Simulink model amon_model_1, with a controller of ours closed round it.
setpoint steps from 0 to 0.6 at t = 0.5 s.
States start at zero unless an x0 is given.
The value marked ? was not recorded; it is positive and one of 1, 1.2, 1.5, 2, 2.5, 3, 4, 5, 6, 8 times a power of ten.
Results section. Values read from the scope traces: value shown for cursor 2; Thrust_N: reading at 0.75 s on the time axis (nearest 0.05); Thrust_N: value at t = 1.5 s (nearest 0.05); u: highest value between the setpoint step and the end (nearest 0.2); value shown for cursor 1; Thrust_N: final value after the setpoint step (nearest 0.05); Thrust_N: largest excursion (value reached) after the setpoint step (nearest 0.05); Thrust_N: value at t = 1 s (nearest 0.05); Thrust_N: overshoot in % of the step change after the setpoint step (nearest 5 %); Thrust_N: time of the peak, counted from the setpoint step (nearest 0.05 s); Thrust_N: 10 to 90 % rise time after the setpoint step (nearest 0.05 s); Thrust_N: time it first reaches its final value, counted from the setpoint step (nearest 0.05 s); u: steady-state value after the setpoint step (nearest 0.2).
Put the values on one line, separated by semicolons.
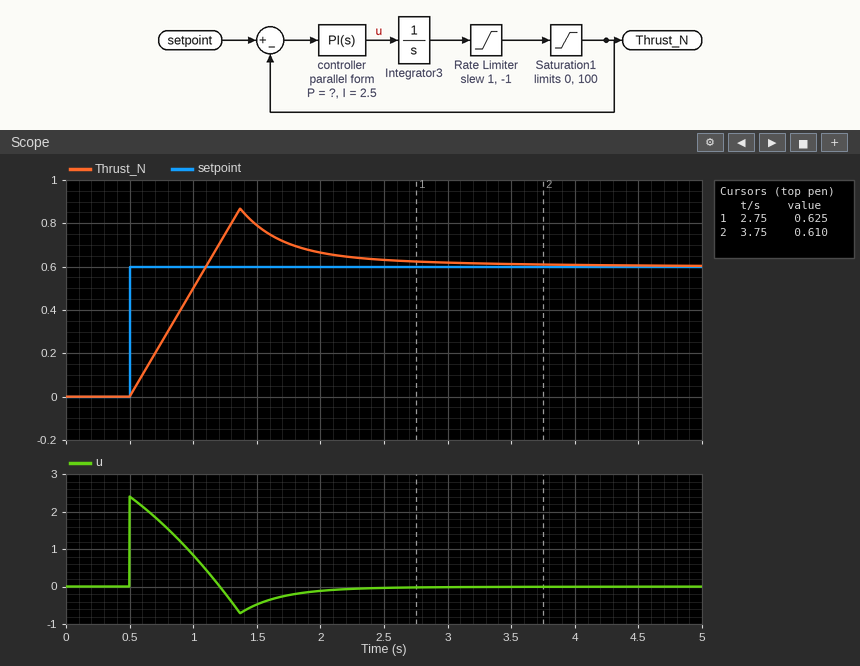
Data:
0.610; 0.25; 0.80; 2.4; 0.625; 0.60; 0.85; 0.50; 45 %; 0.85 s; 0.50 s; 0.60 s; 0.0
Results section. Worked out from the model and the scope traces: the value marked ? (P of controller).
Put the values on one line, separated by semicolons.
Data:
4
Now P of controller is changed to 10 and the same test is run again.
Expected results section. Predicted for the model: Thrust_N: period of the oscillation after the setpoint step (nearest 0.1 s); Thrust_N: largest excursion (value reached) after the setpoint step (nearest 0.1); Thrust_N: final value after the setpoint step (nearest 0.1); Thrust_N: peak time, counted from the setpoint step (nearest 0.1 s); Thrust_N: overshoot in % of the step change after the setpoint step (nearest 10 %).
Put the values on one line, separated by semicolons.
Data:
1.1 s; 1.1; 0.6; 1.1 s; 80 %
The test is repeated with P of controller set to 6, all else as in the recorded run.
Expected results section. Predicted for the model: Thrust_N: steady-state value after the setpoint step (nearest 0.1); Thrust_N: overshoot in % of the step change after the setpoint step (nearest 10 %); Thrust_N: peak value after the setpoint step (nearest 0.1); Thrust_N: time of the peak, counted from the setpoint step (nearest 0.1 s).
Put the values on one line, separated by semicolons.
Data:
0.6; 60 %; 1.0; 1.0 s
